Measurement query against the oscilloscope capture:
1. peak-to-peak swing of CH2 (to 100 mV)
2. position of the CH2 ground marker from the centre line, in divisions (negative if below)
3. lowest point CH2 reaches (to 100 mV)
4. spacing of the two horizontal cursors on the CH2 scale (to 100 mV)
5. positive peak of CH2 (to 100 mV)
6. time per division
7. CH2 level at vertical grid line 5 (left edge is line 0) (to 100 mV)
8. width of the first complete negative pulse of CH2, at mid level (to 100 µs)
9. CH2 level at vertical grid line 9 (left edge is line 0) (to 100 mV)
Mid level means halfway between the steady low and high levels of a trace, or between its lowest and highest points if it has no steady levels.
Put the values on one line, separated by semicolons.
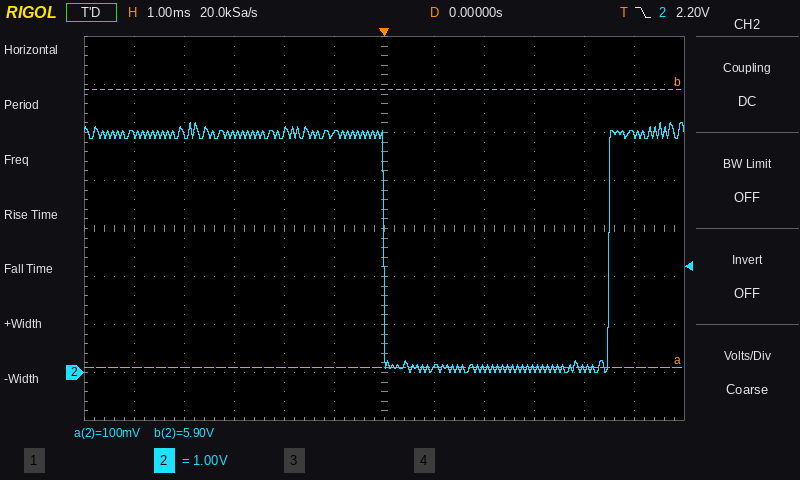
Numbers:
5.2 V; -3.0 div; 0.0 V; 5.8 V; 5.2 V; 1 ms; 5.0 V; 4.5 ms; 100 mV
